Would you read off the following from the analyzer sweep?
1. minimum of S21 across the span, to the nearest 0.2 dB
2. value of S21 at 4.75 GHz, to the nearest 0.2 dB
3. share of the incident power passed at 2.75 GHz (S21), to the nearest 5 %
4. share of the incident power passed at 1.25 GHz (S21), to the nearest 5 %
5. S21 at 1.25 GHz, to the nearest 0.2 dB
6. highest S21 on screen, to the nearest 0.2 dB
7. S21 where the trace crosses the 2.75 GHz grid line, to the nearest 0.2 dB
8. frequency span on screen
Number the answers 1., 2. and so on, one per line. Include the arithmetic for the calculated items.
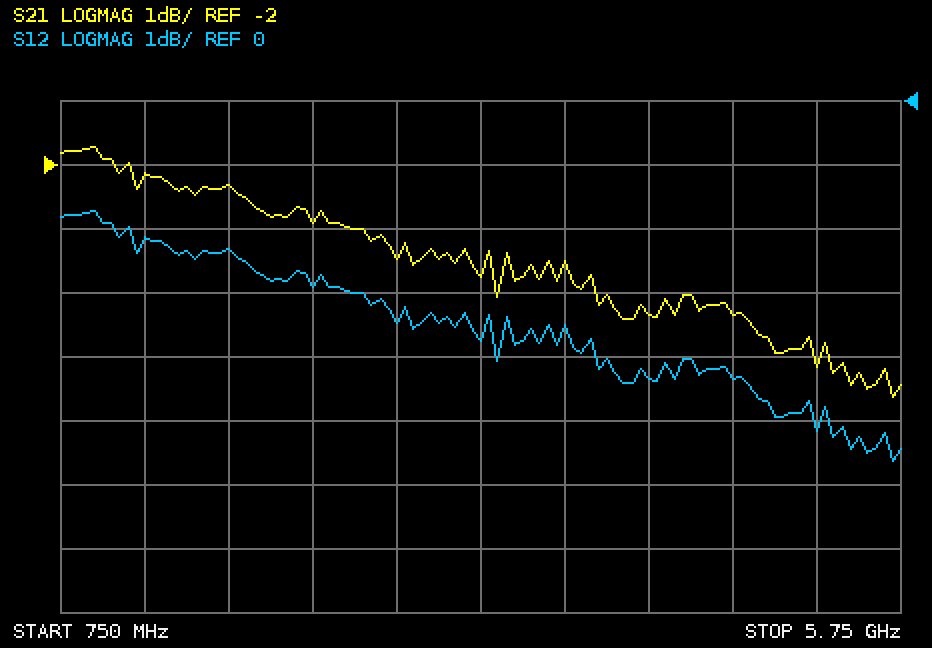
1. -5.6 dB
2. -4.4 dB
3. 10^(-3.4/10) ≈ 45.7 %, so 45 % to the nearest 5 %
4. 10^(-2.2/10) ≈ 60 %
5. -2.2 dB
6. -1.8 dB
7. -3.4 dB
8. 5 GHz
